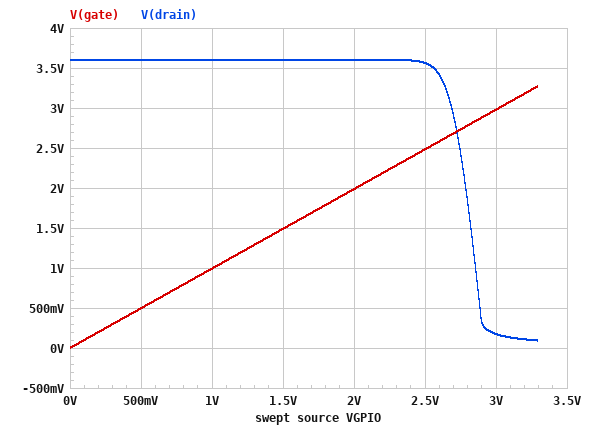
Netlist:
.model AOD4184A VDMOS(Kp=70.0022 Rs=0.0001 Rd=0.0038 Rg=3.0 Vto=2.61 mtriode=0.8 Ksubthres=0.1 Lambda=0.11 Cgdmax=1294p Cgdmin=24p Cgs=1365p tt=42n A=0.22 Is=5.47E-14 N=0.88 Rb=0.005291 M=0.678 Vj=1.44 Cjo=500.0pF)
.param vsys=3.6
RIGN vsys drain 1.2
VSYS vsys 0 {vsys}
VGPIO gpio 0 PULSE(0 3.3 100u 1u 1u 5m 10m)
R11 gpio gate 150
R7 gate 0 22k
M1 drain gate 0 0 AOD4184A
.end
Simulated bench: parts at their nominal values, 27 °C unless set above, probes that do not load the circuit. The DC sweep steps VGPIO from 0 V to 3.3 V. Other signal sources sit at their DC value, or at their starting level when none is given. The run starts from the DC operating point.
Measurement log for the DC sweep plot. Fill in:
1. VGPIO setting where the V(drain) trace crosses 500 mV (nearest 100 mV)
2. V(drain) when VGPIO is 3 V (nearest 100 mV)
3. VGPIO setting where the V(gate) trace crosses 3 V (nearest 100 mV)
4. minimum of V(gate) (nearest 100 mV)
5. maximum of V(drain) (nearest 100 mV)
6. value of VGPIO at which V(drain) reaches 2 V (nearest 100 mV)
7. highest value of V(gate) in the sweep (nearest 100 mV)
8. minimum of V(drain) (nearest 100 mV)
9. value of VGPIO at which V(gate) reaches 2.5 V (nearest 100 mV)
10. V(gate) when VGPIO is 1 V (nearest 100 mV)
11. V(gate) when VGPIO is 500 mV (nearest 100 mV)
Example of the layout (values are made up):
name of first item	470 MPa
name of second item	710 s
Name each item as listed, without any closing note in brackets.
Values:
VGPIO setting where the V(drain) trace crosses 500 mV	2.9 V
V(drain) when VGPIO is 3 V	200 mV
VGPIO setting where the V(gate) trace crosses 3 V	3.0 V
minimum of V(gate)	0 V
maximum of V(drain)	3.6 V
value of VGPIO at which V(drain) reaches 2 V	2.8 V
highest value of V(gate) in the sweep	3.3 V
minimum of V(drain)	100 mV
value of VGPIO at which V(gate) reaches 2.5 V	2.5 V
V(gate) when VGPIO is 1 V	1.0 V
V(gate) when VGPIO is 500 mV	500 mV
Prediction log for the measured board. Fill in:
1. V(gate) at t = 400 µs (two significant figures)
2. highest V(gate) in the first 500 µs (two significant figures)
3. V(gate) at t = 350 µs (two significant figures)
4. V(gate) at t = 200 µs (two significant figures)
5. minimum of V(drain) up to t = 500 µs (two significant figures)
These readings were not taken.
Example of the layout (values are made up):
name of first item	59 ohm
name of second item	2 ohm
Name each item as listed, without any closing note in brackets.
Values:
V(gate) at t = 400 µs	3.3 V
highest V(gate) in the first 500 µs	3.3 V
V(gate) at t = 350 µs	3.3 V
V(gate) at t = 200 µs	3.3 V
minimum of V(drain) up to t = 500 µs	93 mV
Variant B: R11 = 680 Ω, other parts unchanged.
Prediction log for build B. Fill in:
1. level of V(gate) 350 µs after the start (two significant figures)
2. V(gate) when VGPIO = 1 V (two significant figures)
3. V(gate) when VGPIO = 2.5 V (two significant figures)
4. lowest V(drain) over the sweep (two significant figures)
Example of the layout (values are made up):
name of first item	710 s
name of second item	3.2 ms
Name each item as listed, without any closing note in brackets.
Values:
level of V(gate) 350 µs after the start	3.2 V
V(gate) when VGPIO = 1 V	970 mV
V(gate) when VGPIO = 2.5 V	2.4 V
lowest V(drain) over the sweep	100 mV
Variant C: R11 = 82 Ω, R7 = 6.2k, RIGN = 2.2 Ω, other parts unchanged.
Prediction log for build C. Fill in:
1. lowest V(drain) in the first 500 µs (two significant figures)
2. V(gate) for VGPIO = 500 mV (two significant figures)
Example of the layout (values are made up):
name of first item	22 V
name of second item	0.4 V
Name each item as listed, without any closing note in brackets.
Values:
lowest V(drain) in the first 500 µs	52 mV
V(gate) for VGPIO = 500 mV	490 mV
